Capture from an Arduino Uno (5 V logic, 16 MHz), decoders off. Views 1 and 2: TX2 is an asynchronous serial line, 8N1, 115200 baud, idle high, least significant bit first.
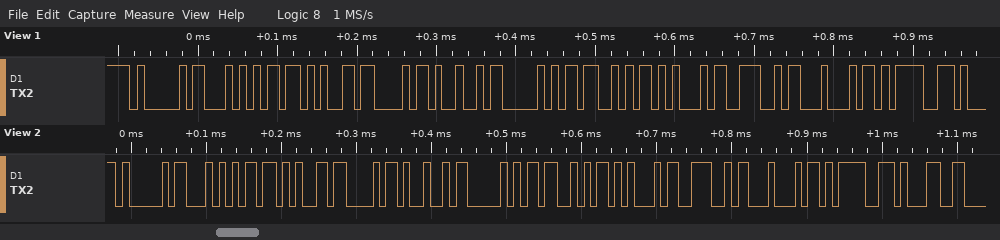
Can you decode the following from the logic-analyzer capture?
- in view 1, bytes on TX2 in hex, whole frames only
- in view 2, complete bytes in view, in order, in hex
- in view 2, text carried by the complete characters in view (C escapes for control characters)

41 54 2B 43 49 50 53 45 4E 44 3D
41 54 2B 43 49 50 53 45 4E 44 3D 31
"AT+CIPSEND=1"
